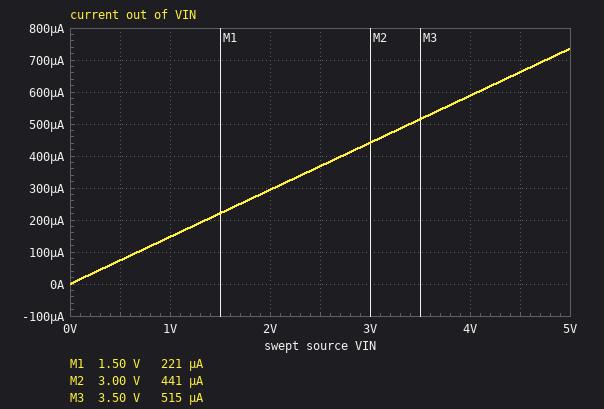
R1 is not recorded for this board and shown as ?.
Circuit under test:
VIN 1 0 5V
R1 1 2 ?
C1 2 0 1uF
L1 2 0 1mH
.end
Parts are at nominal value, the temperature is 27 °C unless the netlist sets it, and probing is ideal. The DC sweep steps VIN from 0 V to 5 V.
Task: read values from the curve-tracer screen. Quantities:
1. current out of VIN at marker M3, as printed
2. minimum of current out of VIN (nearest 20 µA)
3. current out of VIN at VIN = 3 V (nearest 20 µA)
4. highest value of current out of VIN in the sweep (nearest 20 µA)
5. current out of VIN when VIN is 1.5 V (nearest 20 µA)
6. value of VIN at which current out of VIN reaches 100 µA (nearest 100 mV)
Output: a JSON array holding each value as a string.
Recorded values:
["515 µA", "0 A", "440 µA", "740 µA", "220 µA", "700 mV"]
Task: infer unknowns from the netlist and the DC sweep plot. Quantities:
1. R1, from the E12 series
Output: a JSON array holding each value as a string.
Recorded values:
["6.8 kΩ"]
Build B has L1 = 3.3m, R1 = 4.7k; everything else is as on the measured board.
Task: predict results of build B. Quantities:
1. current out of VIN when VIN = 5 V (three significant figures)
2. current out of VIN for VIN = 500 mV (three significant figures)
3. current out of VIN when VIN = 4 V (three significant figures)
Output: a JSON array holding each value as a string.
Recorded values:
["1.06 mA", "106 µA", "851 µA"]
